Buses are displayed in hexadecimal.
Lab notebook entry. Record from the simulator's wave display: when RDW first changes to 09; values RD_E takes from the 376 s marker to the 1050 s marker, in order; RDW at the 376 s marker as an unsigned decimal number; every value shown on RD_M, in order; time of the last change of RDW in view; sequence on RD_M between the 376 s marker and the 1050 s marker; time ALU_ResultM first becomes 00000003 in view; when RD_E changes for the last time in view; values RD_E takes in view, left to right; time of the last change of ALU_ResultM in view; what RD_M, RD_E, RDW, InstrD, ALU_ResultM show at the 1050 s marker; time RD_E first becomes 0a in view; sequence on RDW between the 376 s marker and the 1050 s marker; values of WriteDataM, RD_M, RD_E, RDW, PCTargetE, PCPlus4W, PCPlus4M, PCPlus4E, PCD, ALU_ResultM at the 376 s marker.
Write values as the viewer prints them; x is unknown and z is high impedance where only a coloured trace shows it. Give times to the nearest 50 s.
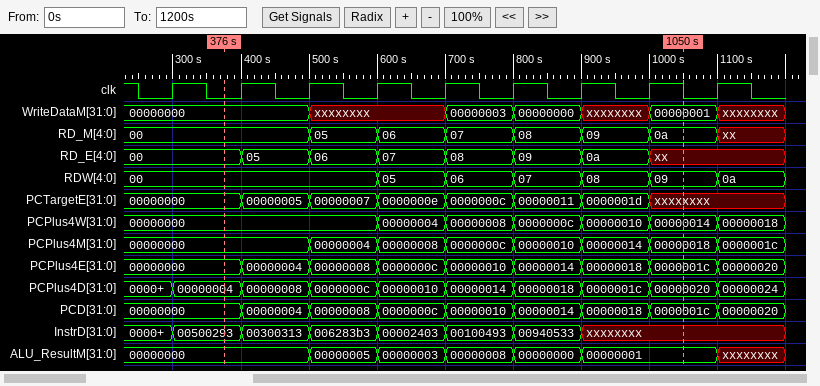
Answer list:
1000 s
00, 05, 06, 07, 08, 09, 0a, xx
0
00, 05, 06, 07, 08, 09, 0a, xx
1100 s
00, 05, 06, 07, 08, 09, 0a
600 s
1000 s
00, 05, 06, 07, 08, 09, 0a, xx
1100 s
RD_M=0a, RD_E=xx, RDW=09, InstrD=xxxxxxxx, ALU_ResultM=00000001
900 s
00, 05, 06, 07, 08, 09
WriteDataM=00000000, RD_M=00, RD_E=00, RDW=00, PCTargetE=00000000, PCPlus4W=00000000, PCPlus4M=00000000, PCPlus4E=00000000, PCD=00000000, ALU_ResultM=00000000
